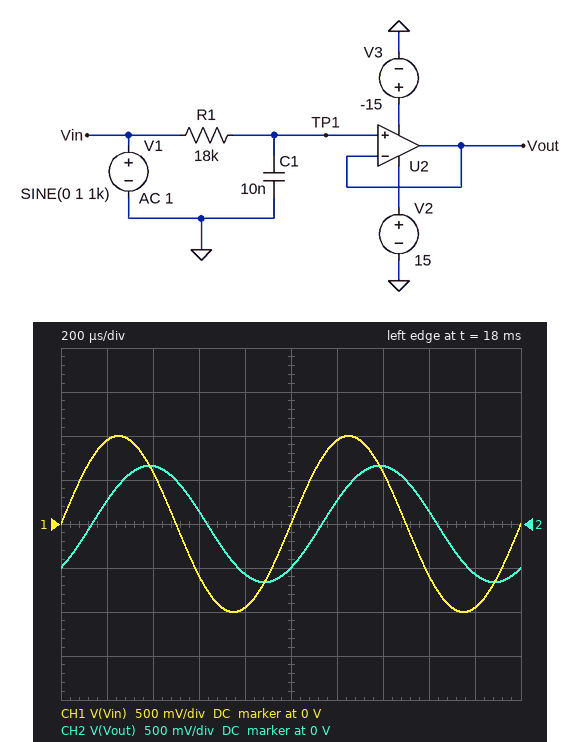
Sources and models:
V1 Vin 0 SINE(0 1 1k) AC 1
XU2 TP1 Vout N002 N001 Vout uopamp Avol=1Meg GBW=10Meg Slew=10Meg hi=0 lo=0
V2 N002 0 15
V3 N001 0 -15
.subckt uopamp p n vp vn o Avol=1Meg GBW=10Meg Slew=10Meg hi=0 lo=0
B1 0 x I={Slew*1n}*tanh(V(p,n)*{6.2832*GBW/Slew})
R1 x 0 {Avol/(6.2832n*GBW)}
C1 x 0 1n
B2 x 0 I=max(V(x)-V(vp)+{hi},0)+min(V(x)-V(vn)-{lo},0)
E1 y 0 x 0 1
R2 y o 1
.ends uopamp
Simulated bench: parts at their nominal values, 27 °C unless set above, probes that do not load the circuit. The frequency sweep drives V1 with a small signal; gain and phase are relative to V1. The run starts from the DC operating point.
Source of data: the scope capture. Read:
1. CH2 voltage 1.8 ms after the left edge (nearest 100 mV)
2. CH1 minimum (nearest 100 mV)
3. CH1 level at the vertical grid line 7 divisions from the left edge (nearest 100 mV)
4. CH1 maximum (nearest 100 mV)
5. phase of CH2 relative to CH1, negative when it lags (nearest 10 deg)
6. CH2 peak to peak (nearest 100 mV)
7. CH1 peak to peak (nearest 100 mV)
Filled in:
-600 mV
-1.0 V
600 mV
1.0 V
-50 deg
1.3 V
2.0 V
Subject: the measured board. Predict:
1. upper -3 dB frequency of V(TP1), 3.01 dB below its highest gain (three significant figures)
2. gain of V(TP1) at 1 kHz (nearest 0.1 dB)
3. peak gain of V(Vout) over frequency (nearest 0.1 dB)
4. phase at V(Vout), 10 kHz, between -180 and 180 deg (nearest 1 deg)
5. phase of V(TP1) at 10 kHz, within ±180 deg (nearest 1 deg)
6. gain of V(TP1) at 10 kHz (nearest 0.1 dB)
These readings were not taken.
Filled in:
884 Hz
-3.6 dB
0 dB
-85 deg
-85 deg
-21.1 dB
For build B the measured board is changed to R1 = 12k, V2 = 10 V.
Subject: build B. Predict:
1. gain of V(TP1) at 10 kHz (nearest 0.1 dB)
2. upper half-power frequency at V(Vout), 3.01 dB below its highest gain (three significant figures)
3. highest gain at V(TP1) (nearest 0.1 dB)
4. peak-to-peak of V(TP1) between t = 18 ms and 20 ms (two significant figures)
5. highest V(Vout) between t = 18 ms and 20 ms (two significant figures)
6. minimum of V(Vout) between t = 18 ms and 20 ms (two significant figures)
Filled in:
-17.6 dB
1.33 kHz
0 dB
1.6 V
800 mV
-800 mV
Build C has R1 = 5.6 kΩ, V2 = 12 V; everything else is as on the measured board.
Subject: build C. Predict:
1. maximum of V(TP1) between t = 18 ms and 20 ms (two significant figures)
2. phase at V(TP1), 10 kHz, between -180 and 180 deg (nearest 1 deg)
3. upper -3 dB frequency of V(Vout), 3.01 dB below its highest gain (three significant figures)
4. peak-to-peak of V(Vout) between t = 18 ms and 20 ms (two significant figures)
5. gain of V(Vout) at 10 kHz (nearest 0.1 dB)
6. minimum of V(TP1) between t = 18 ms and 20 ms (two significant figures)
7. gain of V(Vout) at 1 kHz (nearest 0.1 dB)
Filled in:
940 mV
-74 deg
2.84 kHz
1.9 V
-11.3 dB
-940 mV
-0.5 dB
